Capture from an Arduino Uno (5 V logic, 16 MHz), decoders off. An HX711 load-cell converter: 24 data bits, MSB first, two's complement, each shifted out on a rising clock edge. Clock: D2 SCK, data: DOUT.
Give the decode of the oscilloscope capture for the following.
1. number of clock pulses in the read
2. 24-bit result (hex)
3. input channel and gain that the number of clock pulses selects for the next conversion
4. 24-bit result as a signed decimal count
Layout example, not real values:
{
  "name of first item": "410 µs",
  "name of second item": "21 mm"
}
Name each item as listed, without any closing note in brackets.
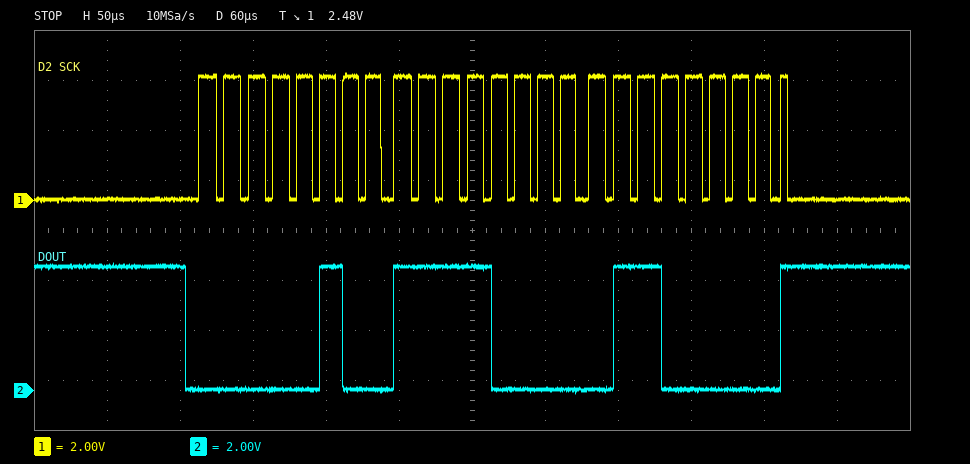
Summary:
{
  "number of clock pulses in the read": "25",
  "24-bit result": "0x04F060",
  "input channel and gain that the number of clock pulses selects for the next conversion": "channel A, gain 128",
  "24-bit result as a signed decimal count": "323680"
}
